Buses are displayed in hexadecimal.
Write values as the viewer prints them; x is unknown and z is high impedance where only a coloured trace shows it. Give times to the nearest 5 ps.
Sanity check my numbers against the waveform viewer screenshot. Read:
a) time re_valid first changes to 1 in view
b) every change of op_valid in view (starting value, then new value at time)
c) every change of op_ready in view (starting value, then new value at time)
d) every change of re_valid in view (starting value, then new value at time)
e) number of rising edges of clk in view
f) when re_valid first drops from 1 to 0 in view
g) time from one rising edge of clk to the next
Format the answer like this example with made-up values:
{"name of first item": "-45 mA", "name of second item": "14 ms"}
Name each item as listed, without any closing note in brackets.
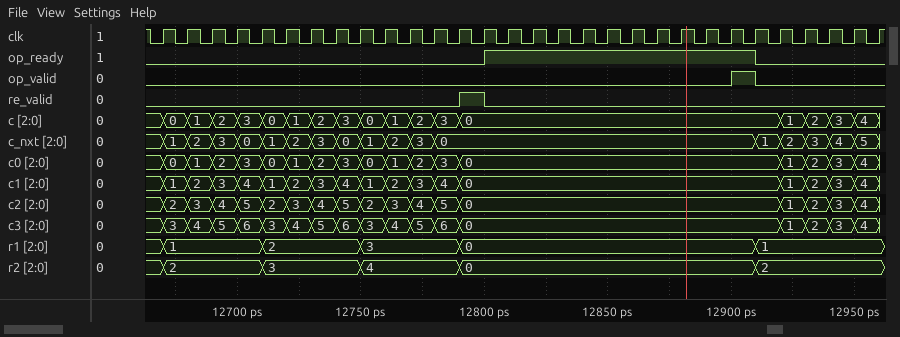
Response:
{"time re_valid first changes to 1 in view": "12790 ps", "every change of op_valid in view": "0, 1 at 12900 ps, 0 at 12910 ps", "every change of op_ready in view": "0, 1 at 12800 ps, 0 at 12910 ps", "every change of re_valid in view": "0, 1 at 12790 ps, 0 at 12800 ps", "number of rising edges of clk in view": "30", "when re_valid first drops from 1 to 0 in view": "12800 ps", "time from one rising edge of clk to the next": "10 ps"}
